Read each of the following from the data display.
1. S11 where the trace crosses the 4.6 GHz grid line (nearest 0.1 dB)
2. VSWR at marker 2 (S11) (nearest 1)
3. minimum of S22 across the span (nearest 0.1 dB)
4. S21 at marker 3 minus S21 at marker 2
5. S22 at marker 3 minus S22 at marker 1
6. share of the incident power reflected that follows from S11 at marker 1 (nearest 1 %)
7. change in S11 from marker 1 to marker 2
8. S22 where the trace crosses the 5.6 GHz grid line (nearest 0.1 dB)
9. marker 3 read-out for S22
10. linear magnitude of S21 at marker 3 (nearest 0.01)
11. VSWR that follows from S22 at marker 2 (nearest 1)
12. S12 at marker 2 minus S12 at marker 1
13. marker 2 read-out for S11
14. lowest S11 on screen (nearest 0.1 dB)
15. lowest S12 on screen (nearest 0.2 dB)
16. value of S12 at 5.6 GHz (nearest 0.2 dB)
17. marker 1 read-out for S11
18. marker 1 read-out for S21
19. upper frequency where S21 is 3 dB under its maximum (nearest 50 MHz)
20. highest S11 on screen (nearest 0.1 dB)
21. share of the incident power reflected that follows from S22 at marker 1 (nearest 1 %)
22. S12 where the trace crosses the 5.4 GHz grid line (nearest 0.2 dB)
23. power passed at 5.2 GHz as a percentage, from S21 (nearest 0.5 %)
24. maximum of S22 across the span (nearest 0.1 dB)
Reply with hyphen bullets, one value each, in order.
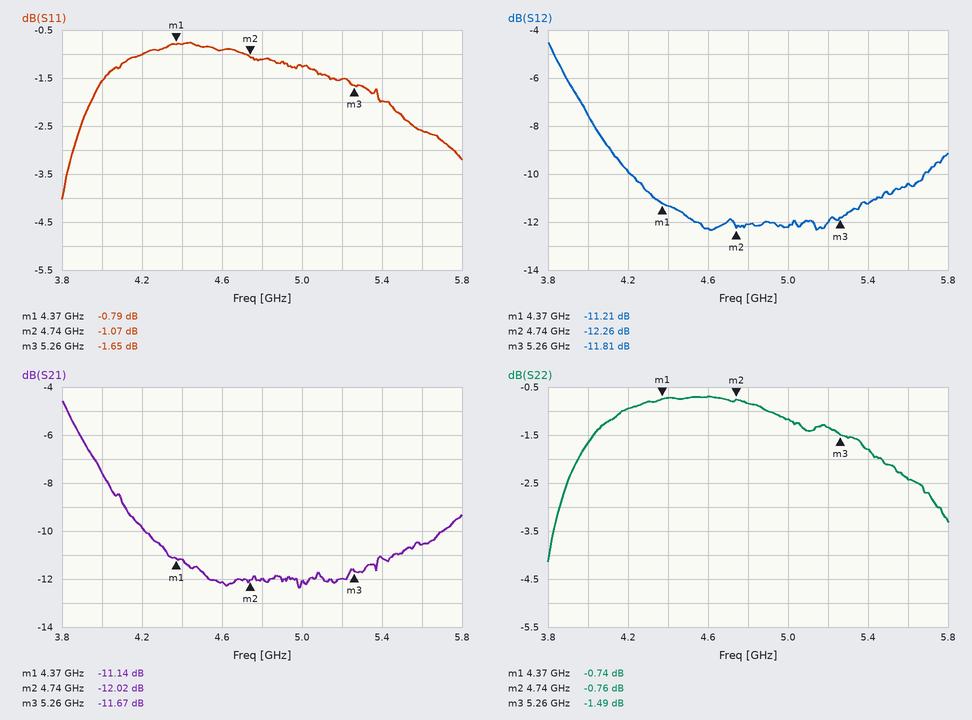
- -0.9 dB
- 16
- -4.1 dB
- 0.35 dB
- -0.75 dB
- 83 %
- -0.28 dB
- -2.4 dB
- -1.49 dB
- 0.26
- 23
- -1.05 dB
- -1.07 dB
- -4.0 dB
- -12.4 dB
- -10.4 dB
- -0.79 dB
- -11.14 dB
- 4.00 GHz
- -0.8 dB
- 84 %
- -11.2 dB
- 6.5 %
- -0.7 dB
